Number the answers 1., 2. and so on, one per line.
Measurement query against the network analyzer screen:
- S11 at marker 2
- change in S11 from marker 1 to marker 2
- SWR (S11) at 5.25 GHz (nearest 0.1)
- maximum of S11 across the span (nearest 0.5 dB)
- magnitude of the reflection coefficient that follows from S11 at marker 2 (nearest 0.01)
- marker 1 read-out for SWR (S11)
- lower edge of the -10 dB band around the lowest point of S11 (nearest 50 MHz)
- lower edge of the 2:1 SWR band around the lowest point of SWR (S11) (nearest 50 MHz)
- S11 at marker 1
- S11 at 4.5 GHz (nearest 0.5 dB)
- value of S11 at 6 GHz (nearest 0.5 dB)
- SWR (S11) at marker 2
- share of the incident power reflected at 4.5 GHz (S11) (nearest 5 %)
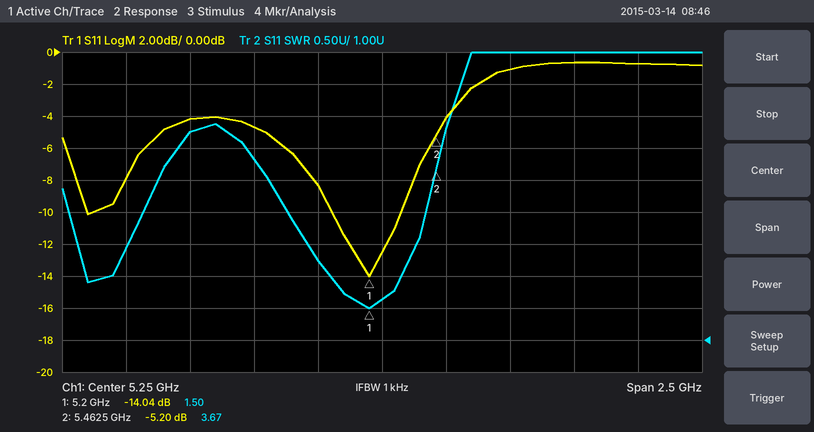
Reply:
1. -5.20 dB
2. 8.84 dB
3. 1.6
4. -0.5 dB
5. 0.55
6. 1.50
7. 5.05 GHz
8. 5.05 GHz
9. -14.04 dB
10. -4.0 dB
11. -0.5 dB
12. 3.67
13. 40 %
